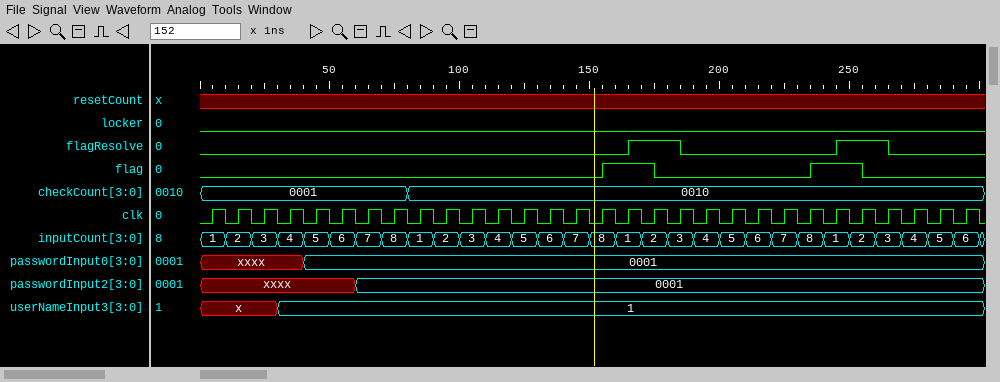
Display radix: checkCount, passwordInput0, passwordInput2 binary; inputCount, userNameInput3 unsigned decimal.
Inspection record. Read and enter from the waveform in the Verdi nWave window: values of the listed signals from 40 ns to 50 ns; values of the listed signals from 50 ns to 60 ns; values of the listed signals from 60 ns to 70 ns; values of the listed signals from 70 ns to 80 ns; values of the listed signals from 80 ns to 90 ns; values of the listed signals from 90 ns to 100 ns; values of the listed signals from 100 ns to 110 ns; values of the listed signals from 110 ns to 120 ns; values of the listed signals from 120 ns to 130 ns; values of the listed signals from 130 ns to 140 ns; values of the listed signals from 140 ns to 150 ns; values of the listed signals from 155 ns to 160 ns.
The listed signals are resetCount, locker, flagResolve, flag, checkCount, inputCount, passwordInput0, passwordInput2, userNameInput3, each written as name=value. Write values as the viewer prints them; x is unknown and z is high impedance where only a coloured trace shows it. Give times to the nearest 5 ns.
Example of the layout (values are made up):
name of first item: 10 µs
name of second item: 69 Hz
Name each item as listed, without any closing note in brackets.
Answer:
values of the listed signals from 40 ns to 50 ns: resetCount=x, locker=0, flagResolve=0, flag=0, checkCount=0001, inputCount=5, passwordInput0=0001, passwordInput2=xxxx, userNameInput3=1
values of the listed signals from 50 ns to 60 ns: resetCount=x, locker=0, flagResolve=0, flag=0, checkCount=0001, inputCount=6, passwordInput0=0001, passwordInput2=xxxx, userNameInput3=1
values of the listed signals from 60 ns to 70 ns: resetCount=x, locker=0, flagResolve=0, flag=0, checkCount=0001, inputCount=7, passwordInput0=0001, passwordInput2=0001, userNameInput3=1
values of the listed signals from 70 ns to 80 ns: resetCount=x, locker=0, flagResolve=0, flag=0, checkCount=0001, inputCount=8, passwordInput0=0001, passwordInput2=0001, userNameInput3=1
values of the listed signals from 80 ns to 90 ns: resetCount=x, locker=0, flagResolve=0, flag=0, checkCount=0010, inputCount=1, passwordInput0=0001, passwordInput2=0001, userNameInput3=1
values of the listed signals from 90 ns to 100 ns: resetCount=x, locker=0, flagResolve=0, flag=0, checkCount=0010, inputCount=2, passwordInput0=0001, passwordInput2=0001, userNameInput3=1
values of the listed signals from 100 ns to 110 ns: resetCount=x, locker=0, flagResolve=0, flag=0, checkCount=0010, inputCount=3, passwordInput0=0001, passwordInput2=0001, userNameInput3=1
values of the listed signals from 110 ns to 120 ns: resetCount=x, locker=0, flagResolve=0, flag=0, checkCount=0010, inputCount=4, passwordInput0=0001, passwordInput2=0001, userNameInput3=1
values of the listed signals from 120 ns to 130 ns: resetCount=x, locker=0, flagResolve=0, flag=0, checkCount=0010, inputCount=5, passwordInput0=0001, passwordInput2=0001, userNameInput3=1
values of the listed signals from 130 ns to 140 ns: resetCount=x, locker=0, flagResolve=0, flag=0, checkCount=0010, inputCount=6, passwordInput0=0001, passwordInput2=0001, userNameInput3=1
values of the listed signals from 140 ns to 150 ns: resetCount=x, locker=0, flagResolve=0, flag=0, checkCount=0010, inputCount=7, passwordInput0=0001, passwordInput2=0001, userNameInput3=1
values of the listed signals from 155 ns to 160 ns: resetCount=x, locker=0, flagResolve=0, flag=1, checkCount=0010, inputCount=8, passwordInput0=0001, passwordInput2=0001, userNameInput3=1
